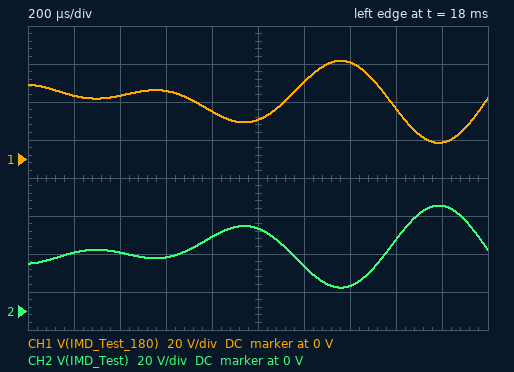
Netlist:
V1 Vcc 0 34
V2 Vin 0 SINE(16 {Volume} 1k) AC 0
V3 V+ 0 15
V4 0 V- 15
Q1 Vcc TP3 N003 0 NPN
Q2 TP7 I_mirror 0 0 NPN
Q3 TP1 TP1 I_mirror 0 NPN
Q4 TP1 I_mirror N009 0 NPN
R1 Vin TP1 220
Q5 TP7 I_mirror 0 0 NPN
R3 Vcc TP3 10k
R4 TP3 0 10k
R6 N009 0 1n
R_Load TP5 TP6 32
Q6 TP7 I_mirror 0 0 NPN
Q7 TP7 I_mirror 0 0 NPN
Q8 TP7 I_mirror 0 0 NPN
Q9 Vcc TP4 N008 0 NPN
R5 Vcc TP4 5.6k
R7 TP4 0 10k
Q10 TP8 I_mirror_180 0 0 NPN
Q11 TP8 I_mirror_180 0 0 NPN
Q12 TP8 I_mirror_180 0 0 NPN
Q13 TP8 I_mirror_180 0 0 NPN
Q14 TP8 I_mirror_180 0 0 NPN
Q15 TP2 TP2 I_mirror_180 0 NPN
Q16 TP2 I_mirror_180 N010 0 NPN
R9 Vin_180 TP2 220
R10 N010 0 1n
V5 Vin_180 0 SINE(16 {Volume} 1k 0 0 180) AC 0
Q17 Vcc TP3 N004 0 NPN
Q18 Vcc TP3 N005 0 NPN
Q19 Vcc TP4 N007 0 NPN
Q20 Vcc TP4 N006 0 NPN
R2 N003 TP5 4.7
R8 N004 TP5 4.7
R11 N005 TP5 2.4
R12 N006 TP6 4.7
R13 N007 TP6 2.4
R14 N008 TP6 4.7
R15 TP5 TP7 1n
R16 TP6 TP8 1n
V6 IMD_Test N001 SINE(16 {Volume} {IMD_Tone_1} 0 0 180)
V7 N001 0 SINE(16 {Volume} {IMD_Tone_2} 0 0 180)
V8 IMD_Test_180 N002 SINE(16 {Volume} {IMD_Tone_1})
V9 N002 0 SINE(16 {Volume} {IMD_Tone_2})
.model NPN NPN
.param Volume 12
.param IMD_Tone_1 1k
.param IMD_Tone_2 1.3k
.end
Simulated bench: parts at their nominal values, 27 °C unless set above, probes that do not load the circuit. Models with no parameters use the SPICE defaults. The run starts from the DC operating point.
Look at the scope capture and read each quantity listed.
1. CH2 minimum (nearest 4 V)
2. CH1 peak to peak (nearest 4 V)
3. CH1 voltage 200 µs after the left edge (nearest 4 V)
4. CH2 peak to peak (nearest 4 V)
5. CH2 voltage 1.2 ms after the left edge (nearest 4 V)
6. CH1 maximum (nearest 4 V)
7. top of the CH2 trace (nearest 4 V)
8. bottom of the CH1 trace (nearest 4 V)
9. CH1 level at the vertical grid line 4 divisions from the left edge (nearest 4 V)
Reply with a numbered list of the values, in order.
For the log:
1. 12 V
2. 44 V
3. 32 V
4. 44 V
5. 24 V
6. 52 V
7. 56 V
8. 8 V
9. 24 V
